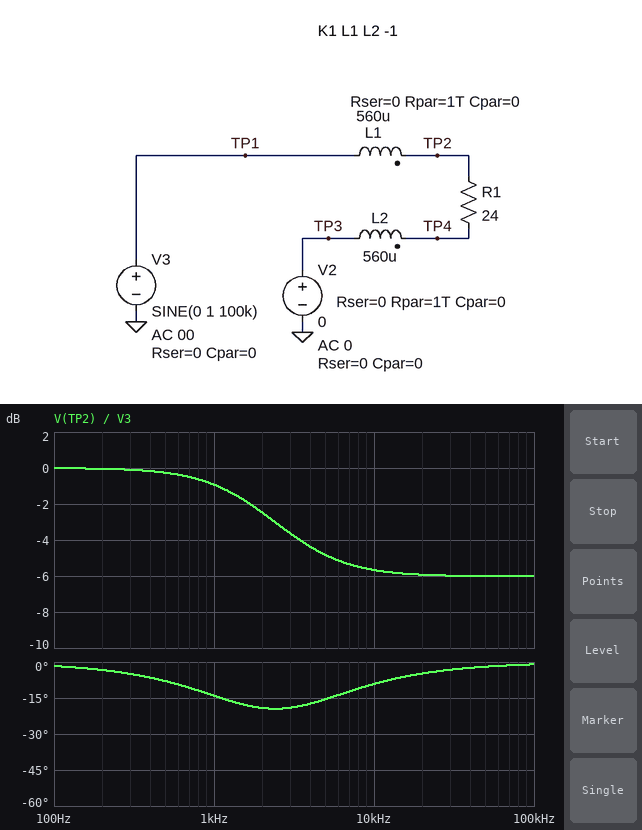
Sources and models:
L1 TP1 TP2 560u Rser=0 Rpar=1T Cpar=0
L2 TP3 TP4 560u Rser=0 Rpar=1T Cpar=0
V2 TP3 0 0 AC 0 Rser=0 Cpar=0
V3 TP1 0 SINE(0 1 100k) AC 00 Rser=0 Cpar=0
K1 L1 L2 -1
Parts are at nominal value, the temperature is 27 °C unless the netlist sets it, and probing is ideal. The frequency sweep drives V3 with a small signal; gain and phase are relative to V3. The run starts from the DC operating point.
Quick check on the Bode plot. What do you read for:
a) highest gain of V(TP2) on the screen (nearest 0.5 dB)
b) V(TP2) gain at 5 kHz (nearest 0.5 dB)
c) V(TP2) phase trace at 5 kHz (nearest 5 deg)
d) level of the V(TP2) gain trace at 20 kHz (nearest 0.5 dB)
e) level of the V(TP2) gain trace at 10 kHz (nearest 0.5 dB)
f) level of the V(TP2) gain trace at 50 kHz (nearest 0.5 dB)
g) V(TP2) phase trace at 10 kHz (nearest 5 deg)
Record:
0 dB
-5.0 dB
-15 deg
-6.0 dB
-5.5 dB
-6.0 dB
-10 deg
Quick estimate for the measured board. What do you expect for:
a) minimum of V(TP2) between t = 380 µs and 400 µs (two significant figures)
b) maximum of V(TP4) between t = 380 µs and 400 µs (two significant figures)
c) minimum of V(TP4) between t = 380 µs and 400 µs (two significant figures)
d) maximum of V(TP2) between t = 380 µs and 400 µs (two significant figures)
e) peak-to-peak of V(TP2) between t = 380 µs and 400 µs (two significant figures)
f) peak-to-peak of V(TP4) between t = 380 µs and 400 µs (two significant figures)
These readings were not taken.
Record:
-500 mV
500 mV
-500 mV
500 mV
1.0 V
1.0 V
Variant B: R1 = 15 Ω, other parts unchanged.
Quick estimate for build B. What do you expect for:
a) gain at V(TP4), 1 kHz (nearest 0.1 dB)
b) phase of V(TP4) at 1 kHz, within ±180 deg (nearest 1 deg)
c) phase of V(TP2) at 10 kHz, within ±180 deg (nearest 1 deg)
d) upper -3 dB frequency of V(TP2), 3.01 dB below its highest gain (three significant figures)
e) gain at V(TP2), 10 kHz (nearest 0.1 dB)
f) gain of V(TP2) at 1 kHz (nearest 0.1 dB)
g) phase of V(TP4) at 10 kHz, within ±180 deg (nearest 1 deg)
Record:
-9.3 dB
47 deg
-6 deg
1.51 kHz
-5.9 dB
-1.9 dB
6 deg
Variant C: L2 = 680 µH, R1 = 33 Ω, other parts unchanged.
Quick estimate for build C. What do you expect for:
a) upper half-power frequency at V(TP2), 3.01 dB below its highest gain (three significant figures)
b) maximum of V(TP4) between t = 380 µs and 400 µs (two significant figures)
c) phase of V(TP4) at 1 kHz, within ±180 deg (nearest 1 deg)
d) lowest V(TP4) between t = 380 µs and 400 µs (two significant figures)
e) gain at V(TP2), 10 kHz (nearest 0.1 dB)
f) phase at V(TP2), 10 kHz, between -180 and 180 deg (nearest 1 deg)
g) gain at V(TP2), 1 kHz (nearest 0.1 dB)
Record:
3.16 kHz
520 mV
65 deg
-520 mV
-5.1 dB
-10 deg
-0.6 dB
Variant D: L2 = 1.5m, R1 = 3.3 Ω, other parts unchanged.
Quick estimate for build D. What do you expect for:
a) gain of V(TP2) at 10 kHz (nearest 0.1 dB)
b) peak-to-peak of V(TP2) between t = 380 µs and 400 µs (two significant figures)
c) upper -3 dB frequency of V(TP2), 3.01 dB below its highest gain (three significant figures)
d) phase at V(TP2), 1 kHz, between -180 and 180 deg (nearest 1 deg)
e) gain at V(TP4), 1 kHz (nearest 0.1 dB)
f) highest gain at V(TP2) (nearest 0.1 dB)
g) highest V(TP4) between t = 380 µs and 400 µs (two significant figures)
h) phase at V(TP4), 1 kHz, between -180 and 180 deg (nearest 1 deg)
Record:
-4.1 dB
1.2 V
282 Hz
-5 deg
-4.2 dB
0 dB
620 mV
8 deg
